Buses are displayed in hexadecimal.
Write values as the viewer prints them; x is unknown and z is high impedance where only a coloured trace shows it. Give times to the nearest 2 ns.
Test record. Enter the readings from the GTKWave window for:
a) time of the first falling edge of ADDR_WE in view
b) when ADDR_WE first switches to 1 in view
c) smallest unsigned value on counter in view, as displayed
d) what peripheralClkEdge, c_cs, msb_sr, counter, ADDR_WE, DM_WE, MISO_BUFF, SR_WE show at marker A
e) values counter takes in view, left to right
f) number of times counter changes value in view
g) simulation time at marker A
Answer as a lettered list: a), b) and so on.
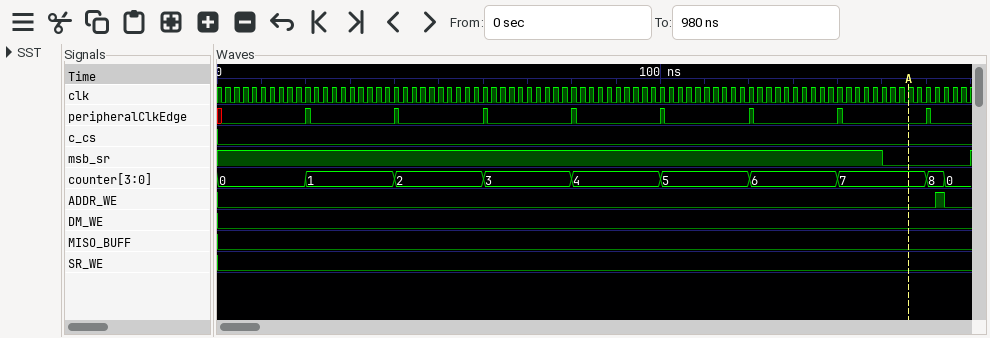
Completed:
a) 164 ns
b) 162 ns
c) 0
d) peripheralClkEdge=0, c_cs=0, msb_sr=0, counter=7, ADDR_WE=0, DM_WE=0, MISO_BUFF=0, SR_WE=0
e) 0, 1, 2, 3, 4, 5, 6, 7, 8, 0
f) 9
g) 156 ns
